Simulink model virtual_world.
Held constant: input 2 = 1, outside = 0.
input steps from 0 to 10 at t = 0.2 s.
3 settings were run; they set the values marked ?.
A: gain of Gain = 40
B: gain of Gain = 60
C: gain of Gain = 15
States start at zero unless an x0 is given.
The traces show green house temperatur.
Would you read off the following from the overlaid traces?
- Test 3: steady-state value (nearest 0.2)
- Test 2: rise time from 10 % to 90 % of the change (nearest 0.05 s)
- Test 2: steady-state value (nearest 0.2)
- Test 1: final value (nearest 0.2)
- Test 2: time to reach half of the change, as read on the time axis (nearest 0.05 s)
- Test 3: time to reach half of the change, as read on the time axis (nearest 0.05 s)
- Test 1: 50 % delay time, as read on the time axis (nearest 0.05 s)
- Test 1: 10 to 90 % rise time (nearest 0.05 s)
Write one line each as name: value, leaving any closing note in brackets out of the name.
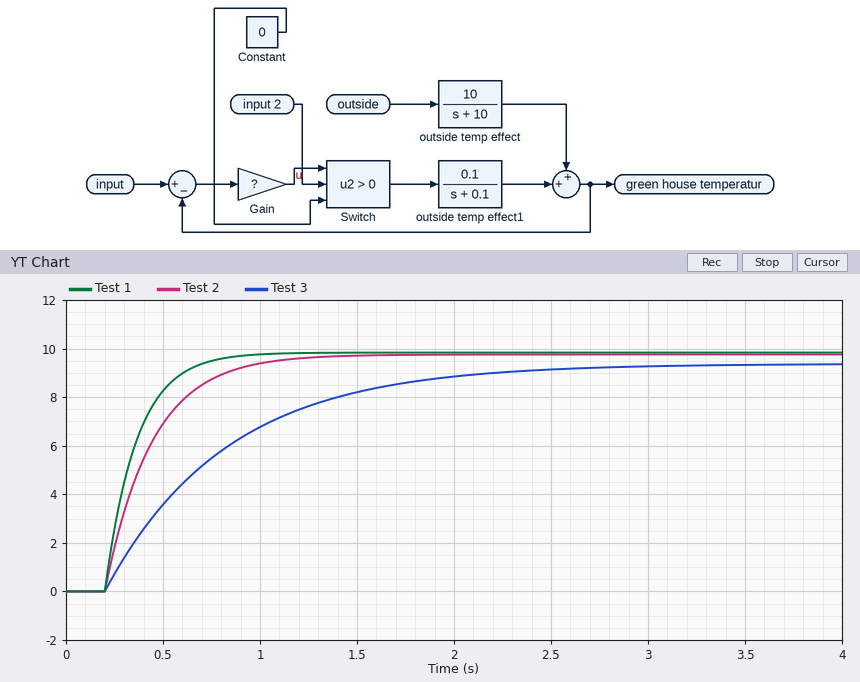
Test 3: steady-state value: 9.4
Test 2: rise time from 10 % to 90 % of the change: 0.55 s
Test 2: steady-state value: 9.8
Test 1: final value: 9.8
Test 2: time to reach half of the change, as read on the time axis: 0.35 s
Test 3: time to reach half of the change, as read on the time axis: 0.65 s
Test 1: 50 % delay time, as read on the time axis: 0.30 s
Test 1: 10 to 90 % rise time: 0.35 s
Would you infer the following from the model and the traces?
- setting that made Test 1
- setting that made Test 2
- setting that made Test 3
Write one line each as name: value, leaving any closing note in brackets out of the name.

setting that made Test 1: B
setting that made Test 2: A
setting that made Test 3: C
